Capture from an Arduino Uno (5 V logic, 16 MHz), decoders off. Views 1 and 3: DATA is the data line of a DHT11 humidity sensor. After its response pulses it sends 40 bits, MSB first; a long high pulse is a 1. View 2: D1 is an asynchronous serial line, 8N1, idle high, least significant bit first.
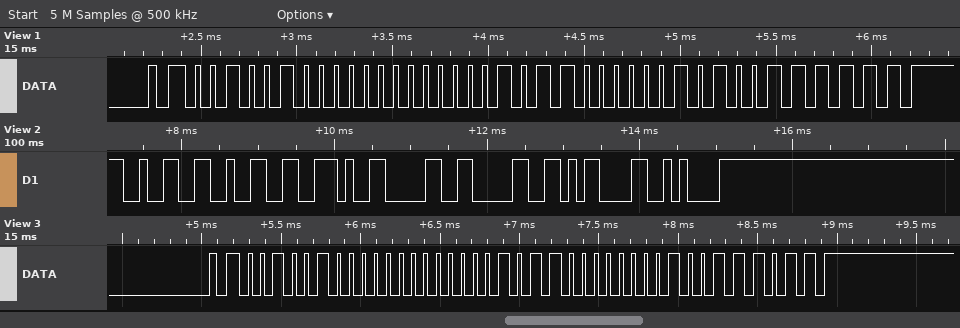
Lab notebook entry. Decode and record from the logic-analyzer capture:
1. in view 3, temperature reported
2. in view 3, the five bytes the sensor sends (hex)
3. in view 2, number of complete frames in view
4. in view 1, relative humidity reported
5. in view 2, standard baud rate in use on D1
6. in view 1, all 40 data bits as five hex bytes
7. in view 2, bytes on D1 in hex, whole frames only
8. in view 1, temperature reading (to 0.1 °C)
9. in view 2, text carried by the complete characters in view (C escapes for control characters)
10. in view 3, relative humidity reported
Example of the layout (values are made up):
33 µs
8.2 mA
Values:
22.1 °C
24 00 16 01 3B
7
36 %
9600 baud
24 00 16 05 3F
0x32 0x32 0x2E 0x30 0x30 0x0D 0x0A
22.5 °C
"22.00\r\n"
36 %
